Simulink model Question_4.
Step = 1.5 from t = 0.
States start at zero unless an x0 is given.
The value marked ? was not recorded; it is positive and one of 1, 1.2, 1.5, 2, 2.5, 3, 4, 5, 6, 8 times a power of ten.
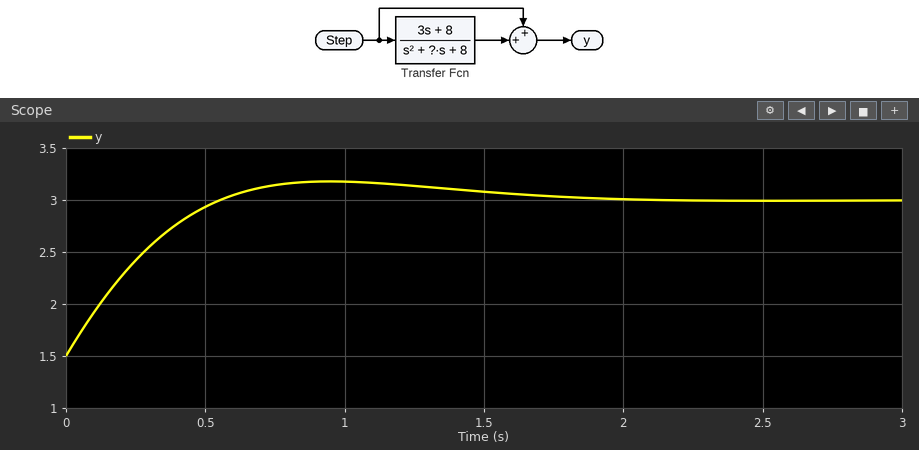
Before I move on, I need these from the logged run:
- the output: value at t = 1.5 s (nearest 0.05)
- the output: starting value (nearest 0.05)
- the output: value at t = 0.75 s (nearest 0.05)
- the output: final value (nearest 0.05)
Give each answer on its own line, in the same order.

3.10
1.50
3.15
3.00
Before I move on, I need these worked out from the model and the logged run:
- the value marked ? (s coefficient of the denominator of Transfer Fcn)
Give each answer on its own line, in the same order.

4
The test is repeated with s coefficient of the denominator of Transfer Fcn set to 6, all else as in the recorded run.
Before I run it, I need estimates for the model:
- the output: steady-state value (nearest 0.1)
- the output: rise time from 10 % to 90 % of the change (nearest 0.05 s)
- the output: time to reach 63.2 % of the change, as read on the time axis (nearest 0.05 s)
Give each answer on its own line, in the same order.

3.0
0.85 s
0.35 s
